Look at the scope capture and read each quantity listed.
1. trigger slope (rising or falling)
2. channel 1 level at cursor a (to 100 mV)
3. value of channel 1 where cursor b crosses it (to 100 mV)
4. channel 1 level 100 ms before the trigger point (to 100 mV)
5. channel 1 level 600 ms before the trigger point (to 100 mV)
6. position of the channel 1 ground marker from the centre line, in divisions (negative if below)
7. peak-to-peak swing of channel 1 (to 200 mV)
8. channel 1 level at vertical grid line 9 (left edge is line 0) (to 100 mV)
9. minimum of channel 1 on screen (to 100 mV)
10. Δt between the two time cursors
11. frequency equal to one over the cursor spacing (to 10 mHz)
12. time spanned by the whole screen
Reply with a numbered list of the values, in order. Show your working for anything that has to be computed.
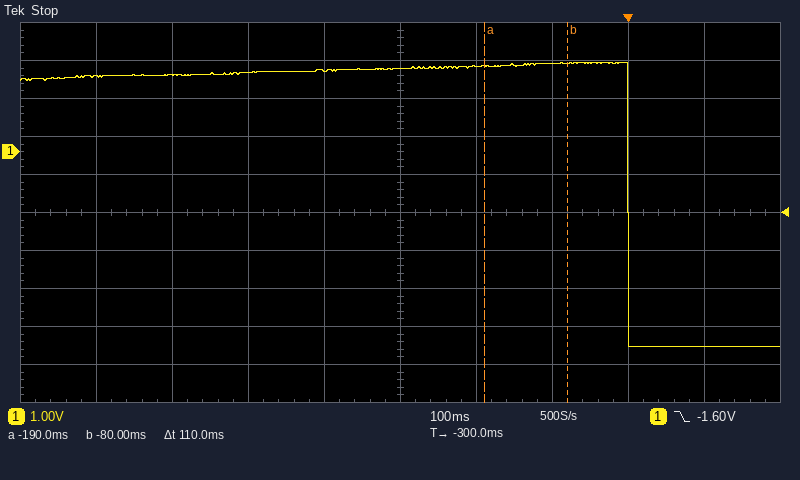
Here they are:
1. falling
2. 2.3 V
3. 2.3 V
4. 2.3 V
5. 2.0 V
6. +1.6 div
7. 7.4 V
8. -5.1 V
9. -5.1 V
10. 110 ms
11. 1 / 110 ms ≈ 9.09 Hz
12. 1 s
